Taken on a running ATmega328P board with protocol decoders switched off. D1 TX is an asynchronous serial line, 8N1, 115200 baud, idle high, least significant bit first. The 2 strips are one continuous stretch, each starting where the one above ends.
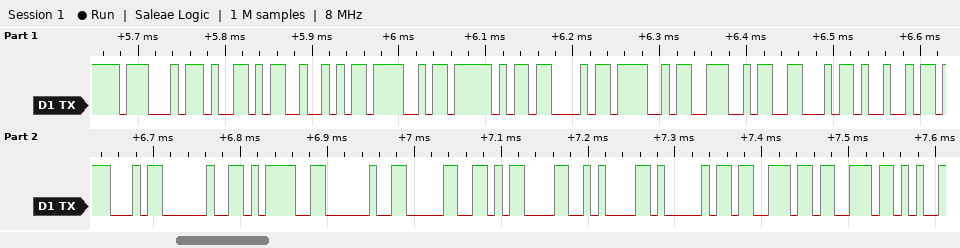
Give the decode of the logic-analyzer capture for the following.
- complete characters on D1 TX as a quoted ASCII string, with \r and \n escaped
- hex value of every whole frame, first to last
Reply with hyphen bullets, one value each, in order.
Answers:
- "GYRO_CONFIG = 0\r\nAss"
- 47 59 52 4F 5F 43 4F 4E 46 49 47 20 3D 20 30 0D 0A 41 73 73
